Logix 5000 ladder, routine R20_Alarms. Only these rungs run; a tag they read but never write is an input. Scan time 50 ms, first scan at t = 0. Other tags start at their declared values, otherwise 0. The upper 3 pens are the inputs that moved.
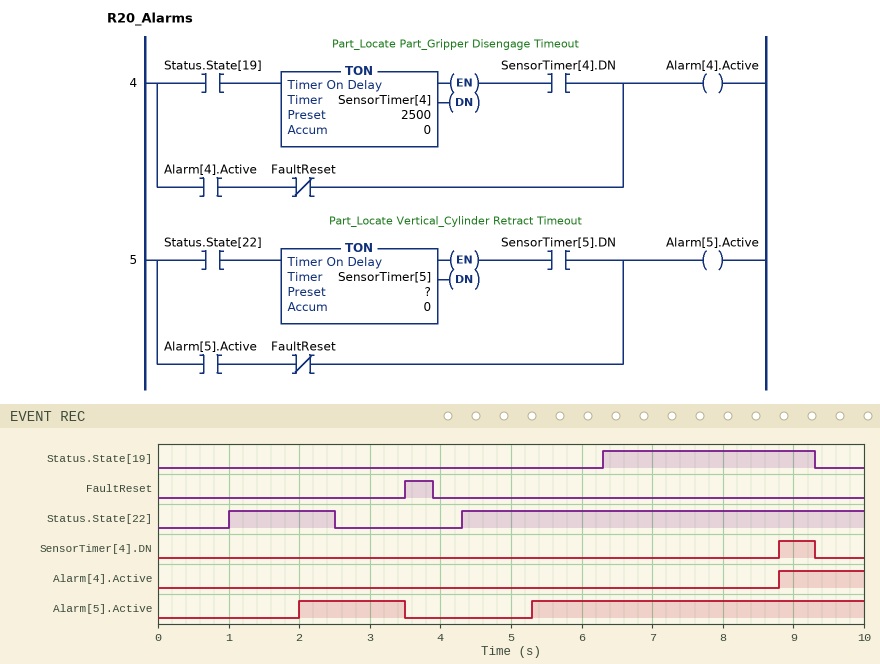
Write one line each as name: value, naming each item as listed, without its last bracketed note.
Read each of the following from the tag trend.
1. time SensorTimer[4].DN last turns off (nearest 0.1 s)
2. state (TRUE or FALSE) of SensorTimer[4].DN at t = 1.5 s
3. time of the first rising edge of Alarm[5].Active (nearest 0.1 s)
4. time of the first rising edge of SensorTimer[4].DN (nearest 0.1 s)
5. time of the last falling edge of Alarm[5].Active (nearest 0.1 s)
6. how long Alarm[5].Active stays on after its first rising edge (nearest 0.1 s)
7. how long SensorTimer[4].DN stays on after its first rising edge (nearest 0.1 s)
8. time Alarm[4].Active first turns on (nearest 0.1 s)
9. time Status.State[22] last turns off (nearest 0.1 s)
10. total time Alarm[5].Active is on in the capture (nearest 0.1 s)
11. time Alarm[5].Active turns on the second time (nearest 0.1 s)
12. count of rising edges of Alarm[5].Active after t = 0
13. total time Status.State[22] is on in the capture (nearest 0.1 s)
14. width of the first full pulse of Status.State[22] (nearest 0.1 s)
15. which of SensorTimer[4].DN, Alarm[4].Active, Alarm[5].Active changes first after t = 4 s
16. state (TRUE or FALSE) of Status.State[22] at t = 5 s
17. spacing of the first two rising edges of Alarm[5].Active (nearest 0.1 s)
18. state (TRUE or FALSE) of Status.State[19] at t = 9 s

time SensorTimer[4].DN last turns off: 9.3 s
state (TRUE or FALSE) of SensorTimer[4].DN at t = 1.5 s: FALSE
time of the first rising edge of Alarm[5].Active: 2.0 s
time of the first rising edge of SensorTimer[4].DN: 8.8 s
time of the last falling edge of Alarm[5].Active: 3.5 s
how long Alarm[5].Active stays on after its first rising edge: 1.5 s
how long SensorTimer[4].DN stays on after its first rising edge: 0.5 s
time Alarm[4].Active first turns on: 8.8 s
time Status.State[22] last turns off: 2.5 s
total time Alarm[5].Active is on in the capture: 6.2 s
time Alarm[5].Active turns on the second time: 5.3 s
count of rising edges of Alarm[5].Active after t = 0: 2
total time Status.State[22] is on in the capture: 7.2 s
width of the first full pulse of Status.State[22]: 1.5 s
which of SensorTimer[4].DN, Alarm[4].Active, Alarm[5].Active changes first after t = 4 s: Alarm[5].Active
state (TRUE or FALSE) of Status.State[22] at t = 5 s: TRUE
spacing of the first two rising edges of Alarm[5].Active: 3.3 s
state (TRUE or FALSE) of Status.State[19] at t = 9 s: TRUE
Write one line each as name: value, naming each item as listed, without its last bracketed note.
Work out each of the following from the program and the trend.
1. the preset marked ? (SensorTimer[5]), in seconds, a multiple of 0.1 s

the preset marked ? (SensorTimer[5]), in seconds, a multiple of 0.1 s: 1.0 s
